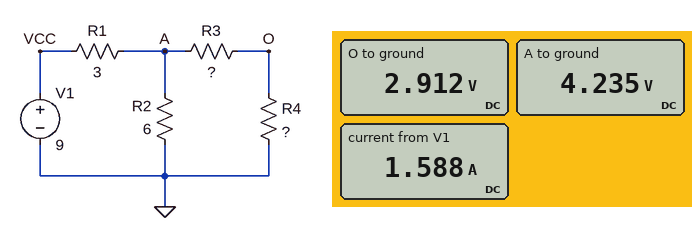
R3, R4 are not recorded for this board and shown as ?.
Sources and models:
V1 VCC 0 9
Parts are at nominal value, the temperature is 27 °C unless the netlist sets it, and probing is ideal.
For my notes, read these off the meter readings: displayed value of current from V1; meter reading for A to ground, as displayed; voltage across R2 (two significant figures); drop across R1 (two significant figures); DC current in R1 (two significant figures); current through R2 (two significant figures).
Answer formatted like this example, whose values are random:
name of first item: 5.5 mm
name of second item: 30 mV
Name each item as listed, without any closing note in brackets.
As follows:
displayed value of current from V1: 1.588 A
meter reading for A to ground, as displayed: 4.235 V
voltage across R2: 4.2 V
drop across R1: 4.8 V
DC current in R1: 1.6 A
current through R2: 710 mA
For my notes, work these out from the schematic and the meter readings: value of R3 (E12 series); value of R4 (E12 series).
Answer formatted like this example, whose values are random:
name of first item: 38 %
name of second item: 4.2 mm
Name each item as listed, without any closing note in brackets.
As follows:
value of R3: 1.5 Ω
value of R4: 3.3 Ω
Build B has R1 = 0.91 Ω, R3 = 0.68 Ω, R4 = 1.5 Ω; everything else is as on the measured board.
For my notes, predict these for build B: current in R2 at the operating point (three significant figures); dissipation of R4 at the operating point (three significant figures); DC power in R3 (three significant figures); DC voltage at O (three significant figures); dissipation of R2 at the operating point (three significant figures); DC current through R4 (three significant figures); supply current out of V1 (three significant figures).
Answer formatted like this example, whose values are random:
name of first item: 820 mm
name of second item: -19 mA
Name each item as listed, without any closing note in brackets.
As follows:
current in R2 at the operating point: 956 mA
dissipation of R4 at the operating point: 10.4 W
DC power in R3: 4.71 W
DC voltage at O: 3.95 V
dissipation of R2 at the operating point: 5.48 W
DC current through R4: 2.63 A
supply current out of V1: 3.59 A
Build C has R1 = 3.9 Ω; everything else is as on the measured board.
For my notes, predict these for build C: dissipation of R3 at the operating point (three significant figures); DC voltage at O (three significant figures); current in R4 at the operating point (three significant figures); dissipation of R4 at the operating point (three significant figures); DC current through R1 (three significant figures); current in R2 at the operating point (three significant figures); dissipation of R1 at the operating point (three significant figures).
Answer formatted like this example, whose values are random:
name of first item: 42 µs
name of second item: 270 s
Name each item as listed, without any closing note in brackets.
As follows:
dissipation of R3 at the operating point: 870 mW
DC voltage at O: 2.51 V
current in R4 at the operating point: 761 mA
dissipation of R4 at the operating point: 1.91 W
DC current through R1: 1.37 A
current in R2 at the operating point: 609 mA
dissipation of R1 at the operating point: 7.33 W
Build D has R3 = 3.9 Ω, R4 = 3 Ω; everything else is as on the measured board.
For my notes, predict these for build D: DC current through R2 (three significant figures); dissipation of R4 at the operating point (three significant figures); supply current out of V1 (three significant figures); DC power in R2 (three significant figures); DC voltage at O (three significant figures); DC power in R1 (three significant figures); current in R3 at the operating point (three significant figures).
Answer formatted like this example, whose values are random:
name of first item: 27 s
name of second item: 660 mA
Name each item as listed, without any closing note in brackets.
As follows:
DC current through R2: 775 mA
dissipation of R4 at the operating point: 1.36 W
supply current out of V1: 1.45 A
DC power in R2: 3.61 W
DC voltage at O: 2.02 V
DC power in R1: 6.30 W
current in R3 at the operating point: 674 mA
